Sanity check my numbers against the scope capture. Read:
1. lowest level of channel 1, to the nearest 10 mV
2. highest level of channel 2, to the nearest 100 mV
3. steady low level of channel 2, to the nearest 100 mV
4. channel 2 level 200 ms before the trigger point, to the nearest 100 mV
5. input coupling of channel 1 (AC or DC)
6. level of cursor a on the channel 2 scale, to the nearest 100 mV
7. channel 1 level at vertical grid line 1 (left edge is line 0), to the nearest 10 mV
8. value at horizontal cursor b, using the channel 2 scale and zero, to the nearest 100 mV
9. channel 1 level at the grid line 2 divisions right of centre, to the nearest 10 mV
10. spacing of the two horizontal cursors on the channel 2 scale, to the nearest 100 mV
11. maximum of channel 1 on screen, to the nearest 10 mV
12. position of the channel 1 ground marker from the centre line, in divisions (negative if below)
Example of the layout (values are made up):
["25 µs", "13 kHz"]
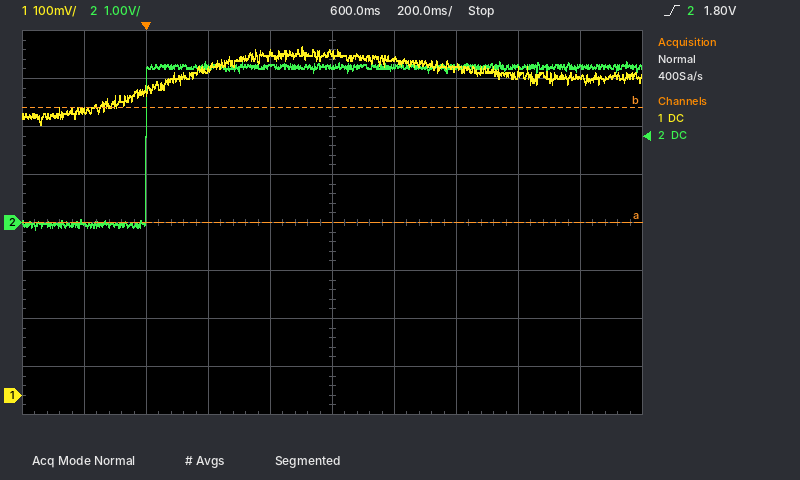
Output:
["560 mV", "3.4 V", "0.0 V", "0.0 V", "DC", "0.0 V", "590 mV", "2.4 V", "680 mV", "2.4 V", "730 mV", "-3.6 div"]
